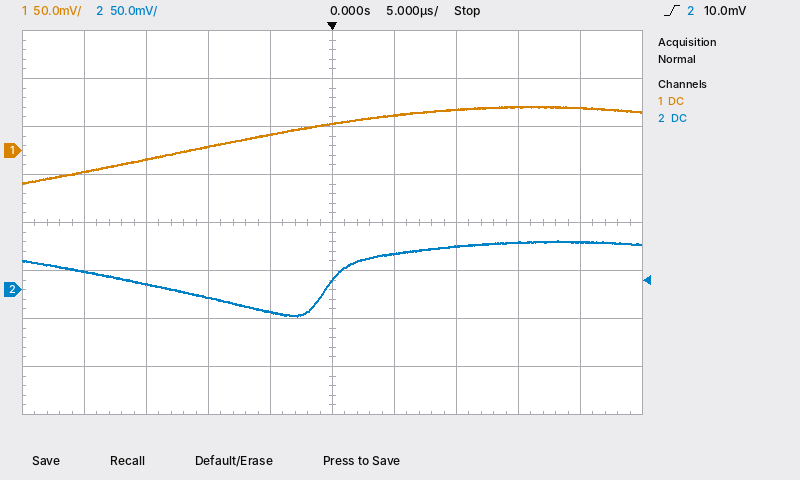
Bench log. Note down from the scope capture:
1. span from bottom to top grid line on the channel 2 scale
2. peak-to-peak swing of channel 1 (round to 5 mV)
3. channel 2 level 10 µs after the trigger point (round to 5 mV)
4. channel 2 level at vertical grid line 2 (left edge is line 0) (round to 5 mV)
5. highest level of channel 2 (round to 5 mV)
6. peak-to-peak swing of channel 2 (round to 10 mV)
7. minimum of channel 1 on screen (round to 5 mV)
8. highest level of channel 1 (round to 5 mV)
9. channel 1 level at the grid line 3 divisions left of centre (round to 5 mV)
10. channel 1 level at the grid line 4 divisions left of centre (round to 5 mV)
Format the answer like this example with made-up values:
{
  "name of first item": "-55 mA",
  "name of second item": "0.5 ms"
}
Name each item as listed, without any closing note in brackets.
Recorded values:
{
  "span from bottom to top grid line on the channel 2 scale": "400 mV",
  "peak-to-peak swing of channel 1": "80 mV",
  "channel 2 level 10 µs after the trigger point": "45 mV",
  "channel 2 level at vertical grid line 2 (left edge is line 0)": "5 mV",
  "highest level of channel 2": "50 mV",
  "peak-to-peak swing of channel 2": "80 mV",
  "minimum of channel 1 on screen": "-35 mV",
  "highest level of channel 1": "45 mV",
  "channel 1 level at the grid line 3 divisions left of centre": "-10 mV",
  "channel 1 level at the grid line 4 divisions left of centre": "-20 mV"
}
